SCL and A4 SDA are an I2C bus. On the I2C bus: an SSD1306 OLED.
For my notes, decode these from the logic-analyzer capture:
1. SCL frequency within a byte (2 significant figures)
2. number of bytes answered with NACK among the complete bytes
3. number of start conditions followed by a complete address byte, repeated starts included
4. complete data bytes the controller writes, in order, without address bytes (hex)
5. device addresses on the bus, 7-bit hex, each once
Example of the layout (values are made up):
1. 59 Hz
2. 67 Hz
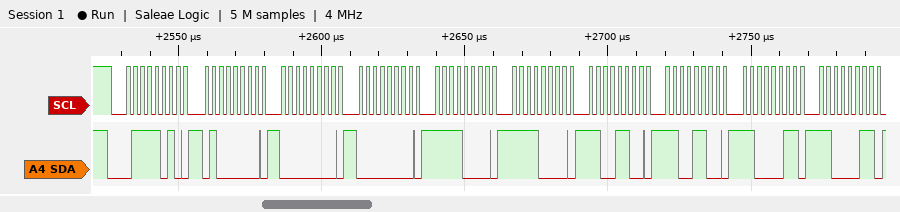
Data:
1. 400 kHz
2. 0
3. 1
4. 40 00 00 F0 F0 CC CC C3 C3
5. 0x3D
